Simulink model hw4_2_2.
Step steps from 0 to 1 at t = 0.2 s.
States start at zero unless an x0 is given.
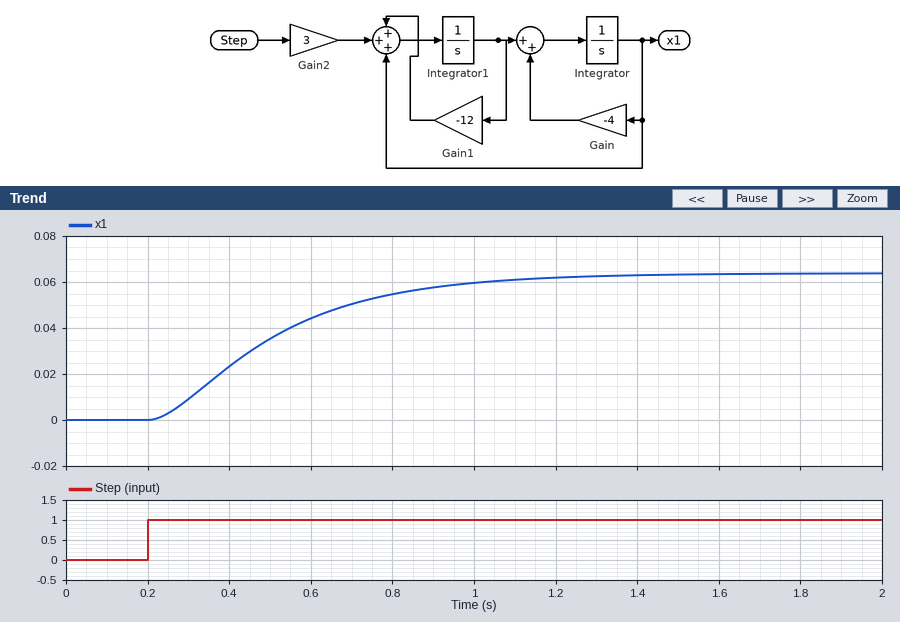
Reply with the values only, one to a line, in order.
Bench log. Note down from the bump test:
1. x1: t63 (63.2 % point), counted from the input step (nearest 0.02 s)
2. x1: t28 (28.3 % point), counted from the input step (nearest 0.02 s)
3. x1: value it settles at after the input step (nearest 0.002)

0.36 s
0.16 s
0.064
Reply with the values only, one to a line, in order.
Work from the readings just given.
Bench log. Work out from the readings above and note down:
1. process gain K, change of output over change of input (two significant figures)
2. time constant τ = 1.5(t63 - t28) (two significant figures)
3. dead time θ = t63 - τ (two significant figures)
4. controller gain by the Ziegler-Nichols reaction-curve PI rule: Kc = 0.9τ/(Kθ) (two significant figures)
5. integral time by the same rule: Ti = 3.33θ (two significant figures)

0.064
0.30 s
0.060 s
70
0.20 s
